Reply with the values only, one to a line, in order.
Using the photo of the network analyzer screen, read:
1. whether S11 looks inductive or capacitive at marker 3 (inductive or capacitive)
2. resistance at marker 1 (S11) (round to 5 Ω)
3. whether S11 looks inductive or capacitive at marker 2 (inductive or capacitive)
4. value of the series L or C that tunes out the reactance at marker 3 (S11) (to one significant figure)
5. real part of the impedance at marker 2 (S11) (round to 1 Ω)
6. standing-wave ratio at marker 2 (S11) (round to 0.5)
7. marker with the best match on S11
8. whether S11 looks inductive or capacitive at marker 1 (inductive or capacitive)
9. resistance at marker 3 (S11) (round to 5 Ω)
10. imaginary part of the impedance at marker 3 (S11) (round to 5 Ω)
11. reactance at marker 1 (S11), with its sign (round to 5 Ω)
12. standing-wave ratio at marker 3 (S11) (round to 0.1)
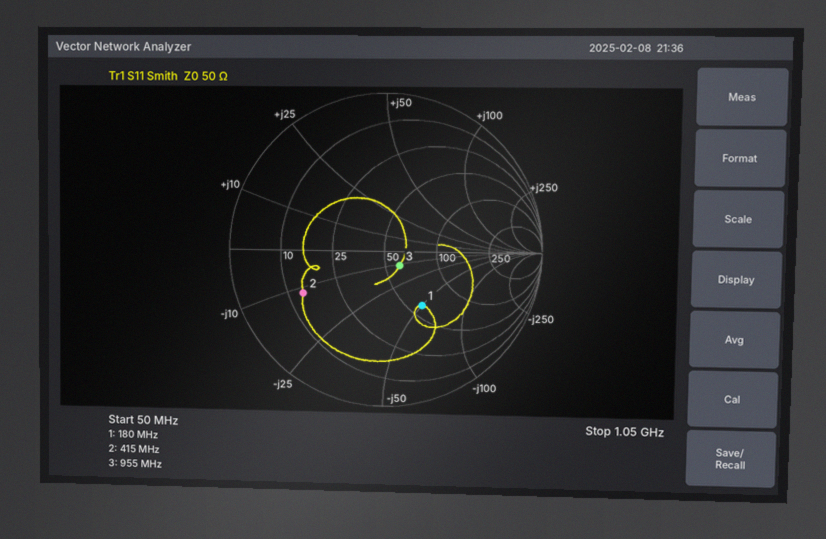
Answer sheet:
capacitive
60 Ω
capacitive
2 nH
14 Ω
4.0
marker 3
capacitive
60 Ω
-10 Ω
-50 Ω
1.3
